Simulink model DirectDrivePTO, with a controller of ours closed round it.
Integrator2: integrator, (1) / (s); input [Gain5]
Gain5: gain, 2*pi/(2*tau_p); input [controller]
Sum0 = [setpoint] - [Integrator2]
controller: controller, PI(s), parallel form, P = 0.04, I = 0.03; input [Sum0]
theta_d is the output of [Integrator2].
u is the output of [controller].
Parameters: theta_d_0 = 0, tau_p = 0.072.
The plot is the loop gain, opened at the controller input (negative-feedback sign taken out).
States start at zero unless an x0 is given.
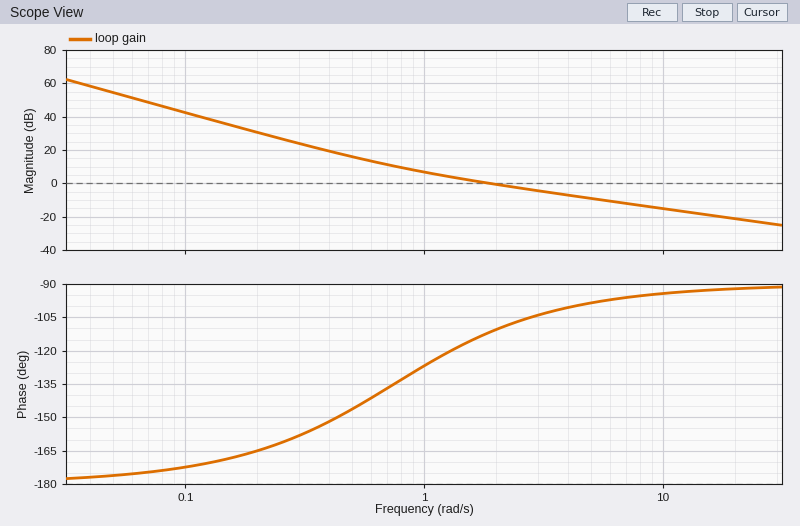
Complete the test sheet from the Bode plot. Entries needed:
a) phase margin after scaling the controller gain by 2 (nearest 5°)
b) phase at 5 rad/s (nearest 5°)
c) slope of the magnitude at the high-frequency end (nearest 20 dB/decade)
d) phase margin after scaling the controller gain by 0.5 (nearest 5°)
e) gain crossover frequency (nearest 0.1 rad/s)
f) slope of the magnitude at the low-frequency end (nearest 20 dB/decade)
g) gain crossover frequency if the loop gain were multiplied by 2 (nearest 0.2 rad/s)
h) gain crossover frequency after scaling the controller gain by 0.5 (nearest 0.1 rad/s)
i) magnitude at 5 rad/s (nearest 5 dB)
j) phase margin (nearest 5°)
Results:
80°
-100°
-20 dB/decade
55°
1.9 rad/s
-40 dB/decade
3.6 rad/s
1.1 rad/s
-10 dB
70°
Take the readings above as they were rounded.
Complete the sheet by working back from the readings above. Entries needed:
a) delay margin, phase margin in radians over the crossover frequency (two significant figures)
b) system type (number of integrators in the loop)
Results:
0.64 s
2
